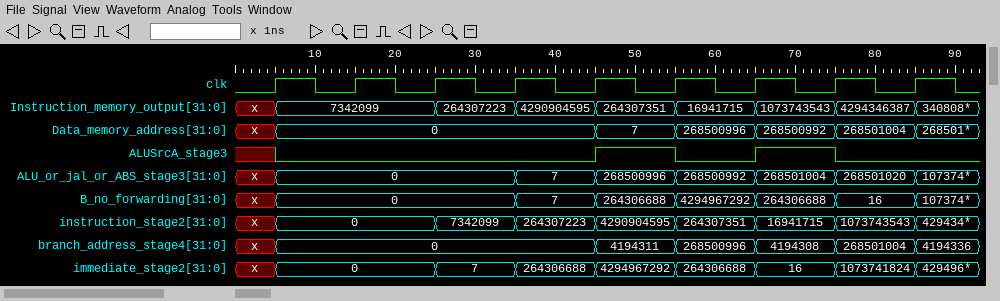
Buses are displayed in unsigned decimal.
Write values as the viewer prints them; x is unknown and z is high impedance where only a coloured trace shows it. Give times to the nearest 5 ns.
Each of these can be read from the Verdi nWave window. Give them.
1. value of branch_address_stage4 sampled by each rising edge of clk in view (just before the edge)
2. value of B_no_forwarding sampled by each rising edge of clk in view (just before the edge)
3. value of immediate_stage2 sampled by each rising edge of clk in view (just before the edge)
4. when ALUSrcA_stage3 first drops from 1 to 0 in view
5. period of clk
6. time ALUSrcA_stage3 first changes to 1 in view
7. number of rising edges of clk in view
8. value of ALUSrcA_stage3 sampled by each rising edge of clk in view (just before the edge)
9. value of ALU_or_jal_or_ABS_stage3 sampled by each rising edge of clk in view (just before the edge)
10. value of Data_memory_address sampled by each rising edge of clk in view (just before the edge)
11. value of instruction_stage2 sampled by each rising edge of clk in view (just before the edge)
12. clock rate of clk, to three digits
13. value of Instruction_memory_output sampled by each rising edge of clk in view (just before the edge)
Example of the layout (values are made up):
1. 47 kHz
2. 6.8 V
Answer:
1. x, 0, 0, 0, 0, 4194311, 268500996, 4194308, 268501004
2. x, 0, 0, 0, 7, 264306688, 4294967292, 264306688, 16
3. x, 0, 0, 7, 264306688, 4294967292, 264306688, 16, 1073741824
4. 55 ns
5. 10 ns
6. 45 ns
7. 9
8. x 0 0 0 0 1 0 1 0
9. x, 0, 0, 0, 7, 268500996, 268500992, 268501004, 268501020
10. x, 0, 0, 0, 0, 7, 268500996, 268500992, 268501004
11. x, 0, 0, 7342099, 264307223, 4290904595, 264307351, 16941715, 1073743543
12. 100 MHz
13. x, 7342099, 7342099, 264307223, 4290904595, 264307351, 16941715, 1073743543, 4294346387
